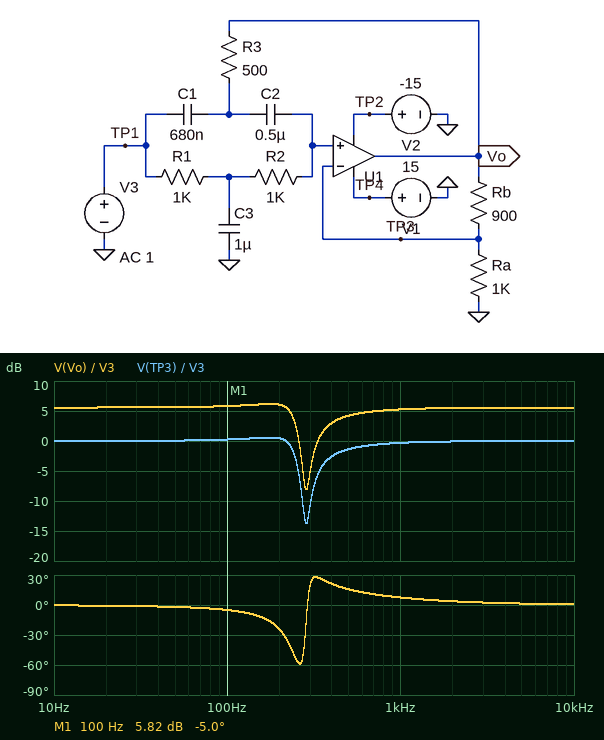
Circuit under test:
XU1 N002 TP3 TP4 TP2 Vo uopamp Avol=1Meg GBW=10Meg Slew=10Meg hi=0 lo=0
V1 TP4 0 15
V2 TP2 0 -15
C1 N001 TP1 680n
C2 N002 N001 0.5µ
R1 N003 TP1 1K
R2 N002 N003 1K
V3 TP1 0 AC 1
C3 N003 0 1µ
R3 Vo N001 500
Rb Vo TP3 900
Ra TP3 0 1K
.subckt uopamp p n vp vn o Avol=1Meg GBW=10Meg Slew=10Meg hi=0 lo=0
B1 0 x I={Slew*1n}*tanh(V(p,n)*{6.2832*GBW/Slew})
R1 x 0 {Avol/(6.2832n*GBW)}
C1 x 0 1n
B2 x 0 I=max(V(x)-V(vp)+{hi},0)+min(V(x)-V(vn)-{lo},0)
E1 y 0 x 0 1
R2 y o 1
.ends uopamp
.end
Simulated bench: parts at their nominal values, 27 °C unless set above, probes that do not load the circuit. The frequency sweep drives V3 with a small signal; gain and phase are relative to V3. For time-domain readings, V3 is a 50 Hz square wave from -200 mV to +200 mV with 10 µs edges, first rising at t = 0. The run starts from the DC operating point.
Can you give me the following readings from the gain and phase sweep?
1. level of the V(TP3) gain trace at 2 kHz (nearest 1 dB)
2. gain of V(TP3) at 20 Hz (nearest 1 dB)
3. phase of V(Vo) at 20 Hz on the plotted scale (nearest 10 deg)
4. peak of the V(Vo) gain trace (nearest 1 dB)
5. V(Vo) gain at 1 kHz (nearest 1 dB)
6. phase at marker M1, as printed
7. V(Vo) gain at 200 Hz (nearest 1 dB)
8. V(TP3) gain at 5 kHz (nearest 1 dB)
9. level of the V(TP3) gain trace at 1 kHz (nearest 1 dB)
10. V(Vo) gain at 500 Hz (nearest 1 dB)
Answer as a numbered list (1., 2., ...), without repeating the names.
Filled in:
1. 0 dB
2. 0 dB
3. 0 deg
4. 6 dB
5. 5 dB
6. -5.0 deg
7. 6 dB
8. 0 dB
9. 0 dB
10. 4 dB
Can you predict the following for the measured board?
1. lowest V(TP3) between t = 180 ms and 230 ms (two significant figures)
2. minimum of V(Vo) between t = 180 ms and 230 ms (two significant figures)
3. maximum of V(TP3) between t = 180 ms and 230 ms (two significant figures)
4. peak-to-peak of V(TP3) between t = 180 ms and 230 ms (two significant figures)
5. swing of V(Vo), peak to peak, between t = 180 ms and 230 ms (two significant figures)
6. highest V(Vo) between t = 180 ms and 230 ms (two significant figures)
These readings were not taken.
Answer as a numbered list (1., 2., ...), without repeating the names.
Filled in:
1. -270 mV
2. -510 mV
3. 270 mV
4. 530 mV
5. 1.0 V
6. 510 mV
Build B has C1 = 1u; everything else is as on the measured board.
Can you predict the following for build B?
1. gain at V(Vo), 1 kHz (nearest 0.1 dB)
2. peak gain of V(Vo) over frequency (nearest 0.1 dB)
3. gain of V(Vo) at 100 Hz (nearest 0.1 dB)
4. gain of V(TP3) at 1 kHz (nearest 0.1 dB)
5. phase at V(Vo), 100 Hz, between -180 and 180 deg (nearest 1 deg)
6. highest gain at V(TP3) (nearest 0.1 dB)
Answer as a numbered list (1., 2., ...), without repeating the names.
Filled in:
1. 5.0 dB
2. 6.7 dB
3. 6.3 dB
4. -0.6 dB
5. -8 deg
6. 1.1 dB
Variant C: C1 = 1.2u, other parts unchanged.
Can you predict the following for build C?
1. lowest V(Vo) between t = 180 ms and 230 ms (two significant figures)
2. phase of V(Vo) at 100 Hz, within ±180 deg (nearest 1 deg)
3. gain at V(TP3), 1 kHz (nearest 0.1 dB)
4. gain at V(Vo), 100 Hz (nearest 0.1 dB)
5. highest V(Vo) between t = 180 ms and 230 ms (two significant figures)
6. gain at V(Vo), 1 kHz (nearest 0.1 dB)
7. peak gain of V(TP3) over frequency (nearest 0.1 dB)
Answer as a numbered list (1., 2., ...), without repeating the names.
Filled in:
1. -520 mV
2. -10 deg
3. -0.7 dB
4. 6.5 dB
5. 520 mV
6. 4.9 dB
7. 1.2 dB
